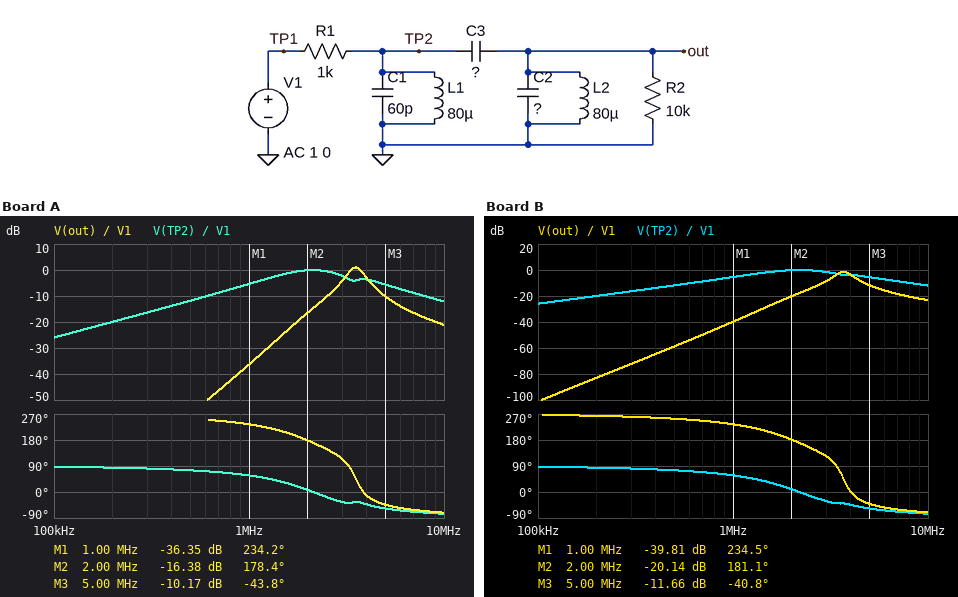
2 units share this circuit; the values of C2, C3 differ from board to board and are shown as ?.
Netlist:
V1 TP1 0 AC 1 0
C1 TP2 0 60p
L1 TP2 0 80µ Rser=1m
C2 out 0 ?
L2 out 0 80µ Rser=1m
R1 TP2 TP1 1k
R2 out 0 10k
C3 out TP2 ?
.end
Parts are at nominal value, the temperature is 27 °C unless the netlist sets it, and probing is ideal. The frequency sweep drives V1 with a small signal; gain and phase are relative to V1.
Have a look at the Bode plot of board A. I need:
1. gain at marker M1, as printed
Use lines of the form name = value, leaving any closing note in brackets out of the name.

gain at marker M1, as printed = -36.35 dB
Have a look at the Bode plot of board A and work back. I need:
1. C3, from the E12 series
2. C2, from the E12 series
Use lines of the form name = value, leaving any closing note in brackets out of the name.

C3, from the E12 series = 8.2 pF
C2, from the E12 series = 18 pF
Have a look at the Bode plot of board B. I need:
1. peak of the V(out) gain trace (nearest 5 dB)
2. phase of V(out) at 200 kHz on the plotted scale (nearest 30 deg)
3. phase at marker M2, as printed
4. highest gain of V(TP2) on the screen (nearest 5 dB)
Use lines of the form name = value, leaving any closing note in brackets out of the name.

peak of the V(out) gain trace = 0 dB
phase of V(out) at 200 kHz on the plotted scale = 270 deg
phase at marker M2, as printed = 181.1 deg
highest gain of V(TP2) on the screen = 0 dB
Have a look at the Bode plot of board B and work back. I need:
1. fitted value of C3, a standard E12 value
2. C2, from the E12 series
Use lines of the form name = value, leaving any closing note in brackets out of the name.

fitted value of C3, a standard E12 value = 5.6 pF
C2, from the E12 series = 18 pF
